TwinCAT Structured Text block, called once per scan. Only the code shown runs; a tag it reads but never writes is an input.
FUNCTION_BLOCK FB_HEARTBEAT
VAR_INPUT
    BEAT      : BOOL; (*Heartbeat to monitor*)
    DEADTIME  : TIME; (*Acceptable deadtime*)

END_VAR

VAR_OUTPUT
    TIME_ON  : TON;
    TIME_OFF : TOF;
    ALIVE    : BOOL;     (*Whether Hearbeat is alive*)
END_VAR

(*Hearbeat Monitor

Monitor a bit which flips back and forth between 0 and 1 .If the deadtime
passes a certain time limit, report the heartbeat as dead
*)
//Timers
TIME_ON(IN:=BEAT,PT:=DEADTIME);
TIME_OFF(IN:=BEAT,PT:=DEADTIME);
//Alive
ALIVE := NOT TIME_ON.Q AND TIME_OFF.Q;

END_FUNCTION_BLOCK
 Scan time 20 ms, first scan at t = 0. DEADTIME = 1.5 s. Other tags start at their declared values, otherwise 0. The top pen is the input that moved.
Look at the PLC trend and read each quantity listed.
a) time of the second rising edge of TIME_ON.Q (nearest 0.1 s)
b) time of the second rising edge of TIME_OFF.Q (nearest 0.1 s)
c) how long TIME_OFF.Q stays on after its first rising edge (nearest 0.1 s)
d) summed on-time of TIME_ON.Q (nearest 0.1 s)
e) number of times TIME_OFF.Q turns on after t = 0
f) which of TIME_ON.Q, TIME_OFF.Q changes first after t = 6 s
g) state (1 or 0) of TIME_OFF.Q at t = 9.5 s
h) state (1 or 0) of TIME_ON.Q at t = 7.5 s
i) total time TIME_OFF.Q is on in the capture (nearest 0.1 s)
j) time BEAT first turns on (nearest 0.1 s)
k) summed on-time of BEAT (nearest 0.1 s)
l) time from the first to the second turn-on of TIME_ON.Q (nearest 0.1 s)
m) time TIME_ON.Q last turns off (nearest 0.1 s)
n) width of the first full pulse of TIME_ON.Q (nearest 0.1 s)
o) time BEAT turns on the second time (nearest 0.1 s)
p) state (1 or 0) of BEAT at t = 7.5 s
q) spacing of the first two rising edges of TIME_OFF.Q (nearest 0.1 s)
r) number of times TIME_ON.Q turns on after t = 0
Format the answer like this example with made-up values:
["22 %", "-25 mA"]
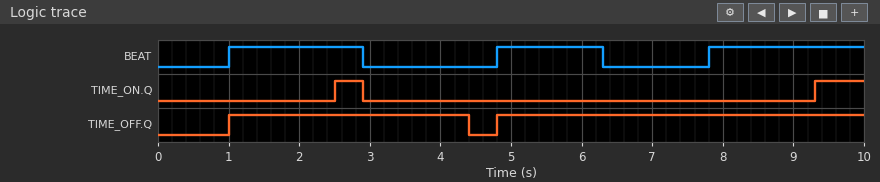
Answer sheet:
["9.3 s", "4.8 s", "3.4 s", "1.1 s", "2", "TIME_ON.Q", "1", "0", "8.6 s", "1.0 s", "5.6 s", "6.8 s", "2.9 s", "0.4 s", "4.8 s", "0", "3.8 s", "2"]
